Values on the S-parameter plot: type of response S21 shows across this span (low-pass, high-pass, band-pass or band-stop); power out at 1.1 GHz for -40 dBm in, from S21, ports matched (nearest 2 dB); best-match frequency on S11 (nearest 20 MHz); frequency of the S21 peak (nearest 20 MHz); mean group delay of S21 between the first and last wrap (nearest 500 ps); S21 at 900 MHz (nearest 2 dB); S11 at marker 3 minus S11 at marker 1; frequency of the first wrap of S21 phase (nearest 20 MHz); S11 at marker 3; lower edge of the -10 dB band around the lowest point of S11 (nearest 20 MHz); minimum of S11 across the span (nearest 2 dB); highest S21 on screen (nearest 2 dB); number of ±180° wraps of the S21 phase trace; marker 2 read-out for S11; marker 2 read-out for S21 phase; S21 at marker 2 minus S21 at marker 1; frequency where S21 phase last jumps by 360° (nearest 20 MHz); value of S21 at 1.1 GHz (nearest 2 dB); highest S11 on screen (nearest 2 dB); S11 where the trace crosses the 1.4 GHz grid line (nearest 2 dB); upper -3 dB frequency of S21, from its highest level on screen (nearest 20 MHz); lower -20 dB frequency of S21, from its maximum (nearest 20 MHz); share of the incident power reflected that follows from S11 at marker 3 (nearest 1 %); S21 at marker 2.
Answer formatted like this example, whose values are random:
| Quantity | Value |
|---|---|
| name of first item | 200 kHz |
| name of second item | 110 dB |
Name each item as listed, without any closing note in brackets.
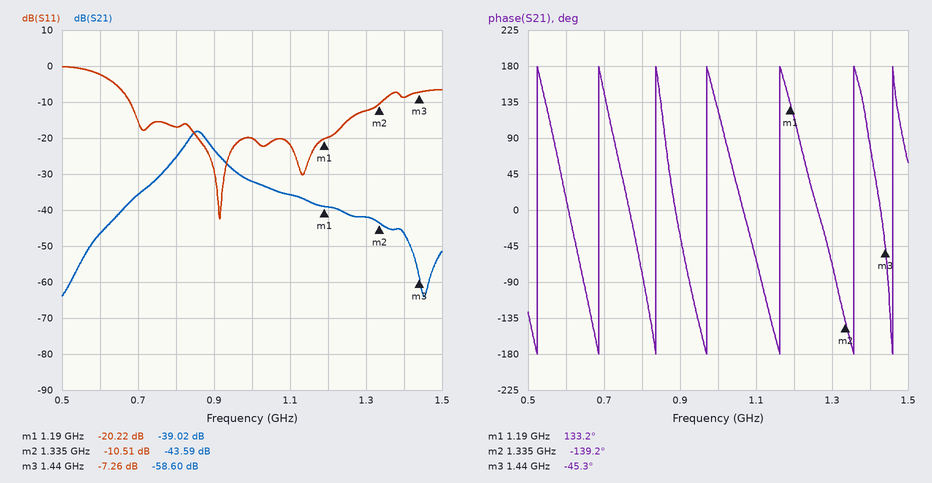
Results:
| Quantity | Value |
|---|---|
| type of response S21 shows across this span | band-pass |
| power out at 1.1 GHz for -40 dBm in, from S21, ports matched | -76 dBm |
| best-match frequency on S11 | 920 MHz |
| frequency of the S21 peak | 860 MHz |
| mean group delay of S21 between the first and last wrap | 6.5 ns |
| S21 at 900 MHz | -24 dB |
| S11 at marker 3 minus S11 at marker 1 | 12.96 dB |
| frequency of the first wrap of S21 phase | 520 MHz |
| S11 at marker 3 | -7.26 dB |
| lower edge of the -10 dB band around the lowest point of S11 | 680 MHz |
| minimum of S11 across the span | -42 dB |
| highest S21 on screen | -18 dB |
| number of ±180° wraps of the S21 phase trace | 7 |
| marker 2 read-out for S11 | -10.51 dB |
| marker 2 read-out for S21 phase | -139.2° |
| S21 at marker 2 minus S21 at marker 1 | -4.57 dB |
| frequency where S21 phase last jumps by 360° | 1.46 GHz |
| value of S21 at 1.1 GHz | -36 dB |
| highest S11 on screen | 0 dB |
| S11 where the trace crosses the 1.4 GHz grid line | -8 dB |
| upper -3 dB frequency of S21, from its highest level on screen | 880 MHz |
| lower -20 dB frequency of S21, from its maximum | 680 MHz |
| share of the incident power reflected that follows from S11 at marker 3 | 19 % |
| S21 at marker 2 | -43.59 dB |
